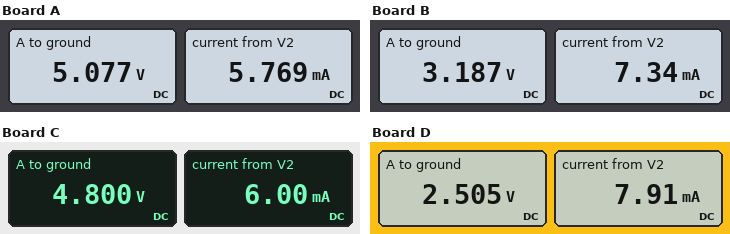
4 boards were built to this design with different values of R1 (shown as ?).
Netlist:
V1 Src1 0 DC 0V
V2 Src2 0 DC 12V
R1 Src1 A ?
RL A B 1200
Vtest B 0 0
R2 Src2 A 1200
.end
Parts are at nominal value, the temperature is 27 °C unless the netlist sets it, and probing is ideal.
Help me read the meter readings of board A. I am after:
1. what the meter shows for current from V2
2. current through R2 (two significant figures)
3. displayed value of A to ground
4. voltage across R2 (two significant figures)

5.769 mA
5.8 mA
5.077 V
6.9 V
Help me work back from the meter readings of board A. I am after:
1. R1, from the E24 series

3.3 kΩ
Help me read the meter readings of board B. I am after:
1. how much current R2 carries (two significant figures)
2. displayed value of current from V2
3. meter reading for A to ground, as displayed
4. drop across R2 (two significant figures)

7.3 mA
7.34 mA
3.187 V
8.8 V
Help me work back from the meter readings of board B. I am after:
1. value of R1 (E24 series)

680 Ω
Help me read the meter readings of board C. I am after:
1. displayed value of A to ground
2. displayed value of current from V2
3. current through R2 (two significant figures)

4.800 V
6.00 mA
6.0 mA
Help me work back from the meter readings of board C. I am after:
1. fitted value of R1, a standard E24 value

2.4 kΩ
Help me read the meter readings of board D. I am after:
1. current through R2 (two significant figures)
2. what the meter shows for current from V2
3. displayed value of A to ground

7.9 mA
7.91 mA
2.505 V
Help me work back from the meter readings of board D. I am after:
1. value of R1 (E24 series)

430 Ω
